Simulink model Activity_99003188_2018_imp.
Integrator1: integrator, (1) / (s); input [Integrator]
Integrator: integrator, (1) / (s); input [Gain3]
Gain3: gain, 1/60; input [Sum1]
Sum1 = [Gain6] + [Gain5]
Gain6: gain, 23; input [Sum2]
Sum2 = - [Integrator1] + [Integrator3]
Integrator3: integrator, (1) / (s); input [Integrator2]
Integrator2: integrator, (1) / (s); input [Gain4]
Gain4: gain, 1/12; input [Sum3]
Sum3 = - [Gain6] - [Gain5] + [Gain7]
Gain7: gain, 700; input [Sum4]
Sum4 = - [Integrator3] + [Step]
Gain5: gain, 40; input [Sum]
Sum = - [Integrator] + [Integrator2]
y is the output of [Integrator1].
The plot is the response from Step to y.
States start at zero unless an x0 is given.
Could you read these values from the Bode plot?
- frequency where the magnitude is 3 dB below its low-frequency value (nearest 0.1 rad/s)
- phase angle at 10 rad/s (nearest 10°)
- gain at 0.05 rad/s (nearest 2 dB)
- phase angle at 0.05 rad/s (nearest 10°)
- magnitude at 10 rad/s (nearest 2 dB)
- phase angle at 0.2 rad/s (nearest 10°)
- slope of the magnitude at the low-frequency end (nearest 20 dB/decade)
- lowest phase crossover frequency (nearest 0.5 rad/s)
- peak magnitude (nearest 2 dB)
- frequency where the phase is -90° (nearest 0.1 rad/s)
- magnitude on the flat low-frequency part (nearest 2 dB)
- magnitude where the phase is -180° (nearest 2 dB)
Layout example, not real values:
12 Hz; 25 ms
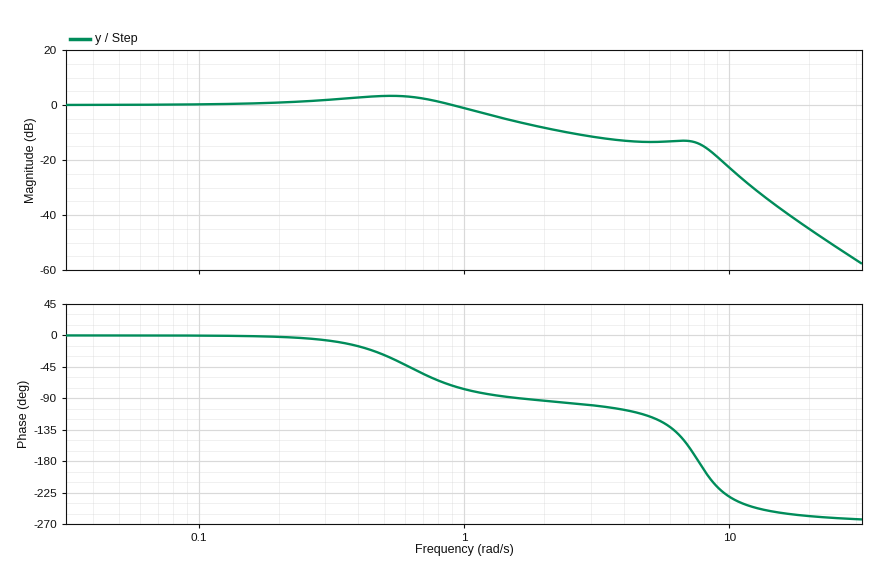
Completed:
1.2 rad/s; -230°; 0 dB; 0°; -22 dB; 0°; 0 dB/decade; 7.5 rad/s; 4 dB; 1.6 rad/s; 0 dB; -14 dB
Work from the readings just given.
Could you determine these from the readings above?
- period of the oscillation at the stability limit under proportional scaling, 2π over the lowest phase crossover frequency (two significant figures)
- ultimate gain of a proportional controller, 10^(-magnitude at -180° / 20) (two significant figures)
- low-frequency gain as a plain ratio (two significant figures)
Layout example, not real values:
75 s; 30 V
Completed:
0.84 s; 5.0; 1.0
